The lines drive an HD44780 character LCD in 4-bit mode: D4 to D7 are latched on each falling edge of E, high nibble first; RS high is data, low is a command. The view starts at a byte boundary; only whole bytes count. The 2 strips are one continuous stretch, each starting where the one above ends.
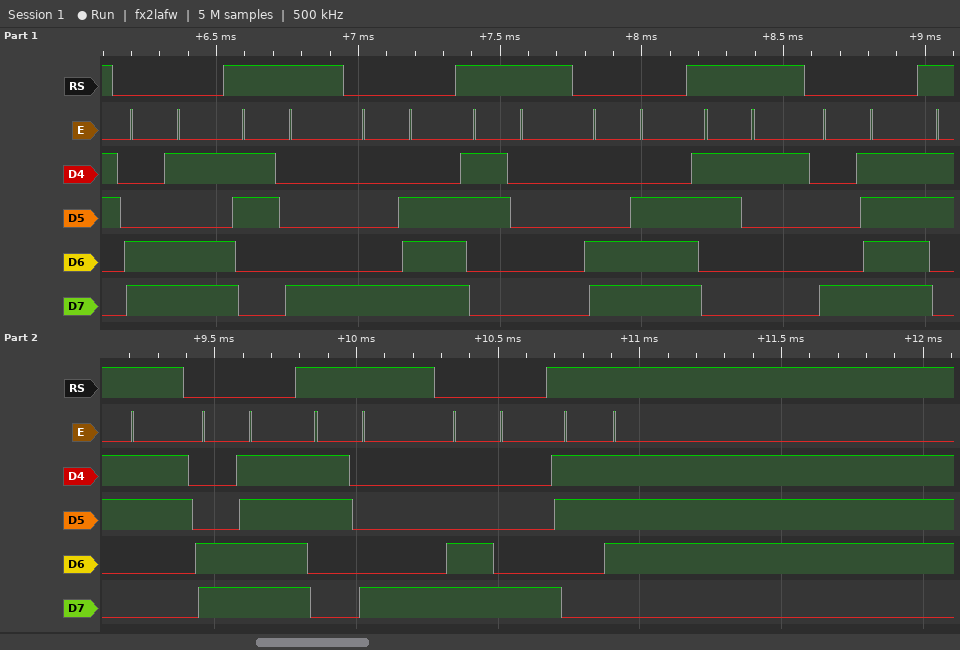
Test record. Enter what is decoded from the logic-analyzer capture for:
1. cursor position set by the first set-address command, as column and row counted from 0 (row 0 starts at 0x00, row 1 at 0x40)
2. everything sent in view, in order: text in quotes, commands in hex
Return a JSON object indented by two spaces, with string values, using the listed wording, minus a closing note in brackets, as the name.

{
  "cursor position set by the first set-address command, as column and row counted from 0": "column 13, row 1",
  "everything sent in view, in order: text in quotes, commands in hex": "0xCD \"8\" 0x8E \"0\" 0xCE \"1\" 0x8F \"3\" 0xCF \"8\" 0xC8 \"7\""
}
